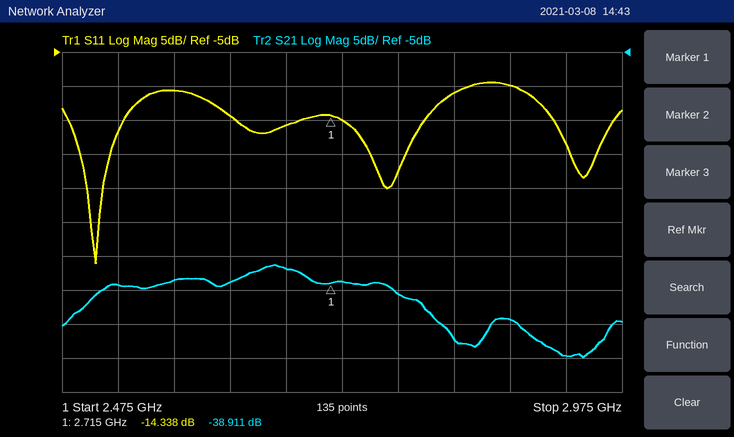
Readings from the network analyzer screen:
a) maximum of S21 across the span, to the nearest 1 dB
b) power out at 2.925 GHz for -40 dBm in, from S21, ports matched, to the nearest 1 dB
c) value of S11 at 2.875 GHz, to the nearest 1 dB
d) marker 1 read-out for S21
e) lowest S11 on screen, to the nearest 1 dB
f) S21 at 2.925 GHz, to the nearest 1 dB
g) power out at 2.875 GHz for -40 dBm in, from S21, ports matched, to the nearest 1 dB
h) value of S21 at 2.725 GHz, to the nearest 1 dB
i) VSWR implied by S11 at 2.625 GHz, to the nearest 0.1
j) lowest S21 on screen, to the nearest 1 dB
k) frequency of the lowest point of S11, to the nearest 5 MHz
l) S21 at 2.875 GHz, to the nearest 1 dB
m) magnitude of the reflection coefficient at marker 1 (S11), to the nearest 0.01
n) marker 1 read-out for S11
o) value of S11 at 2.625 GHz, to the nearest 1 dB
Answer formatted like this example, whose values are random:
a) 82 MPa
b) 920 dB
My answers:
a) -36 dB
b) -90 dBm
c) -10 dB
d) -38.911 dB
e) -36 dB
f) -50 dB
g) -84 dBm
h) -39 dB
i) 1.5
j) -50 dB
k) 2.505 GHz
l) -44 dB
m) 0.19
n) -14.338 dB
o) -14 dB
